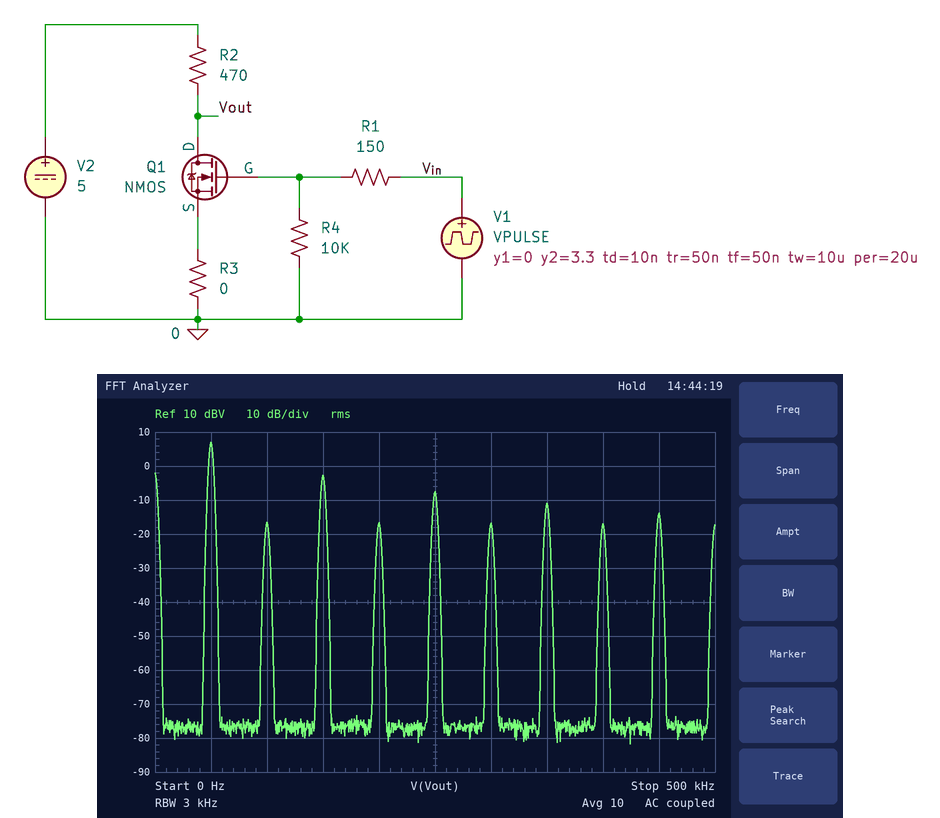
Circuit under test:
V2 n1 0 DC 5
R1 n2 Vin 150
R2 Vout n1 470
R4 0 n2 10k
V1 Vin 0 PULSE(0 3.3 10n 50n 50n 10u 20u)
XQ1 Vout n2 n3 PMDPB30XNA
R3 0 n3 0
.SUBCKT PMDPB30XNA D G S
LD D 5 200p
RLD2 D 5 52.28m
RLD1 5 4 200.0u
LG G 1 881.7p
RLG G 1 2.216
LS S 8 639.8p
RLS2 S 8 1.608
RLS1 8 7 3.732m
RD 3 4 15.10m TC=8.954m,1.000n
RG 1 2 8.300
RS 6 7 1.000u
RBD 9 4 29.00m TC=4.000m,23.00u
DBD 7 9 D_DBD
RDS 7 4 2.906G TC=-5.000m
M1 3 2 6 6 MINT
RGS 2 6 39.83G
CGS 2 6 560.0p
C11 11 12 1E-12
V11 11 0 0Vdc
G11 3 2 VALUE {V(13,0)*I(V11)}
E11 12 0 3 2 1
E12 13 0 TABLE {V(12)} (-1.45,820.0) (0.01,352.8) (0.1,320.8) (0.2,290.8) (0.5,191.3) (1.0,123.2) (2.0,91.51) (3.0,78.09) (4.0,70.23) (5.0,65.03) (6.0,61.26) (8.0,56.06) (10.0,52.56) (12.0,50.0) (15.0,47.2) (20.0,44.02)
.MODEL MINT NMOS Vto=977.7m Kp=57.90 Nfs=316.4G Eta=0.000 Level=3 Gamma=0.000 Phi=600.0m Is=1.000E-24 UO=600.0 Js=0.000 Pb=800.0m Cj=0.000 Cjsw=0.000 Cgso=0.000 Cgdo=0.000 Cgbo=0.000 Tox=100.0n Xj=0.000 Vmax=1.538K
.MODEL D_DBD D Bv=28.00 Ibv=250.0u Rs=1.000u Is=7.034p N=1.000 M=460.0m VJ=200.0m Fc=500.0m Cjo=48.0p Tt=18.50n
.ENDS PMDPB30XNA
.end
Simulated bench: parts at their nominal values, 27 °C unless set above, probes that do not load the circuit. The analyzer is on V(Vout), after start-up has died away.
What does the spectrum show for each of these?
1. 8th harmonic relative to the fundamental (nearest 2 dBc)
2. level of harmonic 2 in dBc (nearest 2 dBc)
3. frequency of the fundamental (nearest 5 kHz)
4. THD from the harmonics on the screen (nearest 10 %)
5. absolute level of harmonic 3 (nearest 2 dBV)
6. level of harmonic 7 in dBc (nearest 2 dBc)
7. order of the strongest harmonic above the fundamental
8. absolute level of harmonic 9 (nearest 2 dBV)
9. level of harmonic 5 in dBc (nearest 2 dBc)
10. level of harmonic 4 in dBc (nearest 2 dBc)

-24 dBc
-24 dBc
50 kHz
40 %
-2 dBV
-18 dBc
3
-14 dBV
-14 dBc
-24 dBc
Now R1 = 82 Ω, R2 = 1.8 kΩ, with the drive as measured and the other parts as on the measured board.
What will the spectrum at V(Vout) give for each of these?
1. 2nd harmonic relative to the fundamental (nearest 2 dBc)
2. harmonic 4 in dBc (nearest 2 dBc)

-22 dBc
-22 dBc
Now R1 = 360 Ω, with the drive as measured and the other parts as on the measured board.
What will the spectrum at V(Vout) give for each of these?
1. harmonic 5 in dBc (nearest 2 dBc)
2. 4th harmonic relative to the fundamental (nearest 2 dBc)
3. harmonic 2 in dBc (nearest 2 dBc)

-16 dBc
-18 dBc
-18 dBc
